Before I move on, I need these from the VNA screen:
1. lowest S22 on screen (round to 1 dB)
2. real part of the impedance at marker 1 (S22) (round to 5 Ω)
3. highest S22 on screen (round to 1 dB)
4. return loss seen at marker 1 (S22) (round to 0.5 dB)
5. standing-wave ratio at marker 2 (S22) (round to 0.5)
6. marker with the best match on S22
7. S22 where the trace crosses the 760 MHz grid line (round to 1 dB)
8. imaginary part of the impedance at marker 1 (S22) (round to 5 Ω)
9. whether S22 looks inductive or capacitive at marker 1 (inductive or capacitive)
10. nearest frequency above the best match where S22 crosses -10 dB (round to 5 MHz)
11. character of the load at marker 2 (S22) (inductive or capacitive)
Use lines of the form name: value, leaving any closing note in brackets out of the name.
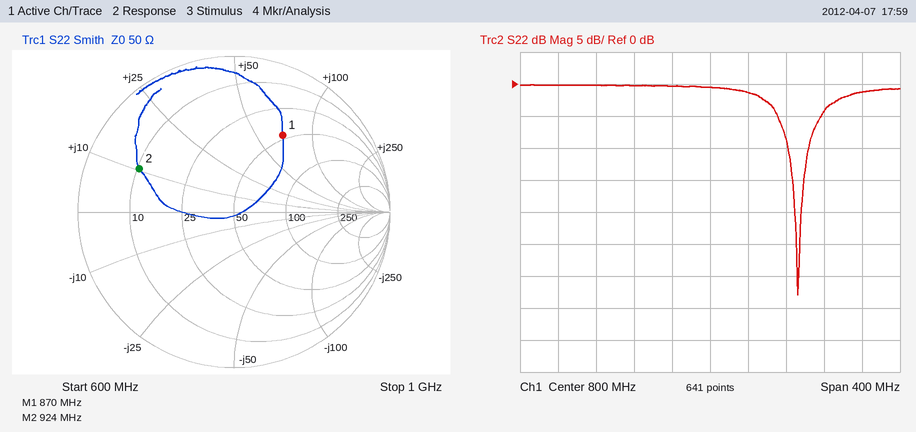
lowest S22 on screen: -33 dB
real part of the impedance at marker 1 (S22): 45 Ω
highest S22 on screen: 0 dB
return loss seen at marker 1 (S22): 4.5 dB
standing-wave ratio at marker 2 (S22): 5.0
marker with the best match on S22: marker 1
S22 where the trace crosses the 760 MHz grid line: 0 dB
imaginary part of the impedance at marker 1 (S22): +70 Ω
whether S22 looks inductive or capacitive at marker 1: inductive
nearest frequency above the best match where S22 crosses -10 dB: 905 MHz
character of the load at marker 2 (S22): inductive
